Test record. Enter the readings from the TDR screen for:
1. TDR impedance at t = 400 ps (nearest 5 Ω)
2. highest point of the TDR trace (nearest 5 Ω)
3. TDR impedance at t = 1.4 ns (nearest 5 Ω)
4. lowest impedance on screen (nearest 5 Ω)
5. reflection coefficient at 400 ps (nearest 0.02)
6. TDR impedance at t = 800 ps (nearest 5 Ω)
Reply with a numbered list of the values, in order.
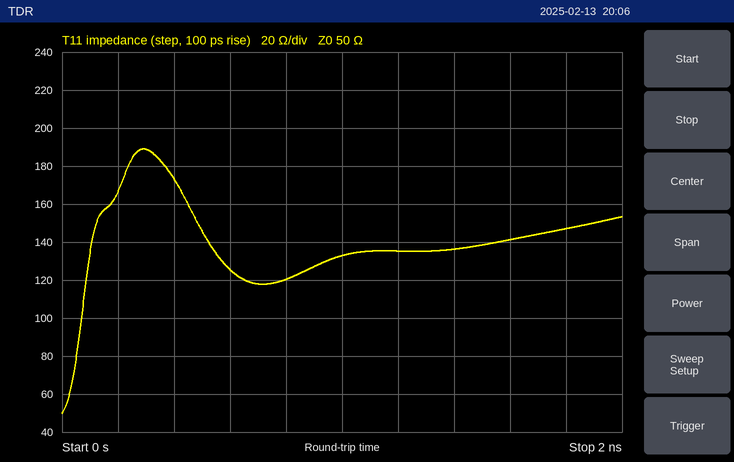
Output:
1. 175 Ω
2. 190 Ω
3. 135 Ω
4. 50 Ω
5. +0.56
6. 120 Ω
